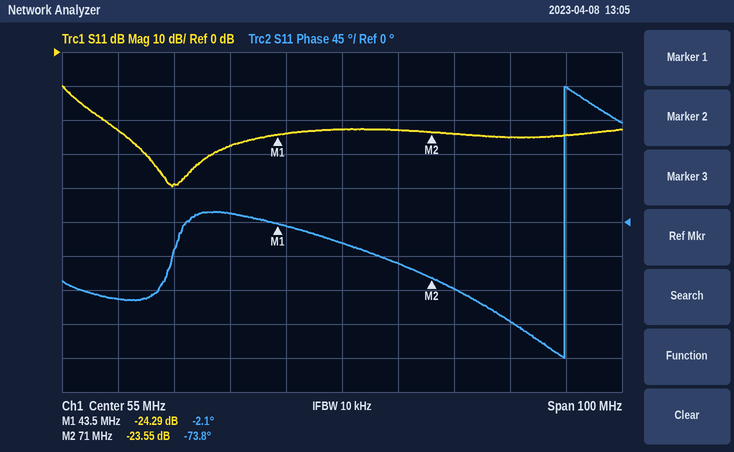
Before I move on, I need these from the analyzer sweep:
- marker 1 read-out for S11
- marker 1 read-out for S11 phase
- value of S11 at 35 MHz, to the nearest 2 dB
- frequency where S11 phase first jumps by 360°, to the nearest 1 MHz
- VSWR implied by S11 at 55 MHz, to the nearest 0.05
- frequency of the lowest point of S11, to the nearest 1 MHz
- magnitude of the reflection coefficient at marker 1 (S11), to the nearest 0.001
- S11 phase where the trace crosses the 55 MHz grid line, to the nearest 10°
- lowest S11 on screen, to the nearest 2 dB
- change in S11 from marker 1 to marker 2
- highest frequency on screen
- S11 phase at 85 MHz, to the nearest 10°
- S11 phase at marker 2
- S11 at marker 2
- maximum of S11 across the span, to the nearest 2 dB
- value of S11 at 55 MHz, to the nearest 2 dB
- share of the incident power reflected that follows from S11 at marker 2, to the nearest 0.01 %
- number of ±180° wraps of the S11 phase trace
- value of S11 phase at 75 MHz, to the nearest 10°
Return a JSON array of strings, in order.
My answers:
["-24.29 dB", "-2.1°", "-28 dB", "95 MHz", "1.15", "25 MHz", "0.061", "-30°", "-40 dB", "0.74 dB", "105 MHz", "-130°", "-73.8°", "-23.55 dB", "-10 dB", "-22 dB", "0.44 %", "1", "-90°"]
